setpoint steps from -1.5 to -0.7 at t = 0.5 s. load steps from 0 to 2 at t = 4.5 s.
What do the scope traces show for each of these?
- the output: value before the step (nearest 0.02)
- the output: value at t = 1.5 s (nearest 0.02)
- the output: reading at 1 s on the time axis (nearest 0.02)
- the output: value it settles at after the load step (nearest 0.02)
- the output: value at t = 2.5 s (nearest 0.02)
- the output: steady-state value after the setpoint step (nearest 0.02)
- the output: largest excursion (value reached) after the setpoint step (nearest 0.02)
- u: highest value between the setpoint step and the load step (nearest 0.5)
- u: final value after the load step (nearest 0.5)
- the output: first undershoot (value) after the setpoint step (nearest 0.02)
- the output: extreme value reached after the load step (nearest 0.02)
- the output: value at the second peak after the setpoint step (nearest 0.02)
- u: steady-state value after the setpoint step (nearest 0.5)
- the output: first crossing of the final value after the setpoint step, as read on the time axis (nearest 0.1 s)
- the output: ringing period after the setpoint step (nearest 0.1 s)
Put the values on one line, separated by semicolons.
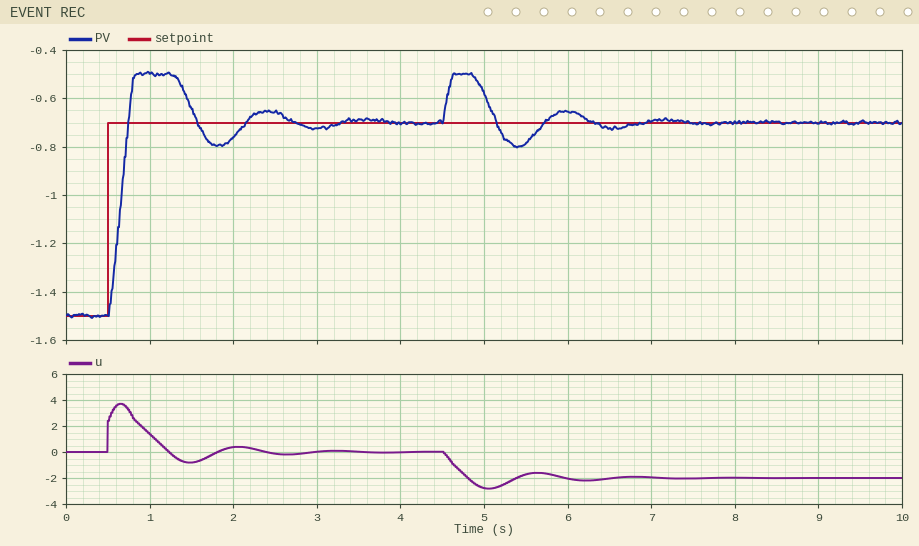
-1.50; -0.64; -0.50; -0.70; -0.66; -0.70; -0.50; 3.5; -2.0; -0.80; -0.50; -0.66; 0.0; 0.7 s; 1.4 s
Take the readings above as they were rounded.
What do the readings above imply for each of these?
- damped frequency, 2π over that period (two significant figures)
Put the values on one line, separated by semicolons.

4.5 rad/s
